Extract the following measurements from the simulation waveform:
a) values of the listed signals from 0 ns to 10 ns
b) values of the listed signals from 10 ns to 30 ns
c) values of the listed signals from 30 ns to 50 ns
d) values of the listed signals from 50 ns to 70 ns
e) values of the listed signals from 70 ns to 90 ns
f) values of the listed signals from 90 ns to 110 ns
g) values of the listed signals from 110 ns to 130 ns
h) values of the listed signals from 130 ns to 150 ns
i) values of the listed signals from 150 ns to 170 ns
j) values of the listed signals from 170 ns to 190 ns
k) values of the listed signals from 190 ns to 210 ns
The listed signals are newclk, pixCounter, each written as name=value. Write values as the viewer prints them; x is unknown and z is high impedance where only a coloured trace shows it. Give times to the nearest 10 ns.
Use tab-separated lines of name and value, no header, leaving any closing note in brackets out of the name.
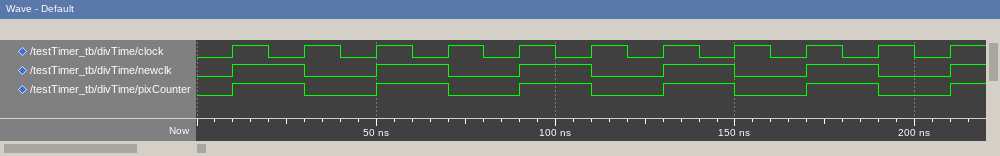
values of the listed signals from 0 ns to 10 ns	newclk=0, pixCounter=0
values of the listed signals from 10 ns to 30 ns	newclk=1, pixCounter=1
values of the listed signals from 30 ns to 50 ns	newclk=0, pixCounter=0
values of the listed signals from 50 ns to 70 ns	newclk=1, pixCounter=1
values of the listed signals from 70 ns to 90 ns	newclk=0, pixCounter=0
values of the listed signals from 90 ns to 110 ns	newclk=1, pixCounter=1
values of the listed signals from 110 ns to 130 ns	newclk=0, pixCounter=0
values of the listed signals from 130 ns to 150 ns	newclk=1, pixCounter=1
values of the listed signals from 150 ns to 170 ns	newclk=0, pixCounter=0
values of the listed signals from 170 ns to 190 ns	newclk=1, pixCounter=1
values of the listed signals from 190 ns to 210 ns	newclk=0, pixCounter=0
